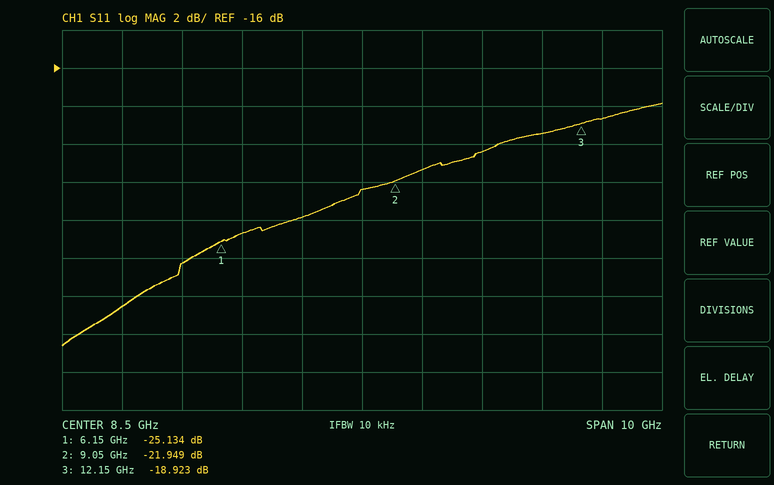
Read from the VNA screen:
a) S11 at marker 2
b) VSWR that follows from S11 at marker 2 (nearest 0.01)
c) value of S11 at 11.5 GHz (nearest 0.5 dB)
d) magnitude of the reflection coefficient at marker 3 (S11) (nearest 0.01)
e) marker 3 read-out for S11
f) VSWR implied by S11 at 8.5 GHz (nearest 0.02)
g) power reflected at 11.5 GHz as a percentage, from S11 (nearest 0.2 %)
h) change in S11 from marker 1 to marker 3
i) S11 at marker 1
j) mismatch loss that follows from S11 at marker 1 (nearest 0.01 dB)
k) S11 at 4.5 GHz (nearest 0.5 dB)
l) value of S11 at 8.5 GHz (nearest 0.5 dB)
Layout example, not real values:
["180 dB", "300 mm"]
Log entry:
["-21.949 dB", "1.17", "-19.5 dB", "0.11", "-18.923 dB", "1.16", "1.2 %", "6.211 dB", "-25.134 dB", "0.01 dB", "-28.5 dB", "-22.5 dB"]
